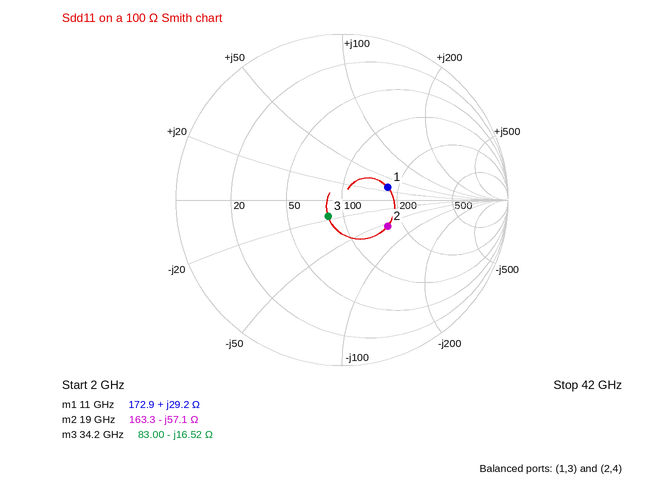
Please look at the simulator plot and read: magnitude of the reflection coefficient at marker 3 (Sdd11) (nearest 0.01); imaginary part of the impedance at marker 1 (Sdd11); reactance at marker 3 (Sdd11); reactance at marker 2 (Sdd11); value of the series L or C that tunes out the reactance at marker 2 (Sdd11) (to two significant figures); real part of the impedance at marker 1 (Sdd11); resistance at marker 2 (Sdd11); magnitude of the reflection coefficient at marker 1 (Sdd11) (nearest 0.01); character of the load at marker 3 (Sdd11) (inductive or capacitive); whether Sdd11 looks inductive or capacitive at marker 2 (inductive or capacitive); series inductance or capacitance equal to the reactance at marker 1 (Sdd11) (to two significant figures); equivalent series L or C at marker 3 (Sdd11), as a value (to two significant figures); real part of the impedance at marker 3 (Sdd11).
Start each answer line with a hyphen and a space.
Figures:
- 0.13
- +29.2 Ω
- -16.52 Ω
- -57.1 Ω
- 480 pH
- 172.9 Ω
- 163.3 Ω
- 0.29
- capacitive
- capacitive
- 420 pH
- 280 fF
- 83.00 Ω
